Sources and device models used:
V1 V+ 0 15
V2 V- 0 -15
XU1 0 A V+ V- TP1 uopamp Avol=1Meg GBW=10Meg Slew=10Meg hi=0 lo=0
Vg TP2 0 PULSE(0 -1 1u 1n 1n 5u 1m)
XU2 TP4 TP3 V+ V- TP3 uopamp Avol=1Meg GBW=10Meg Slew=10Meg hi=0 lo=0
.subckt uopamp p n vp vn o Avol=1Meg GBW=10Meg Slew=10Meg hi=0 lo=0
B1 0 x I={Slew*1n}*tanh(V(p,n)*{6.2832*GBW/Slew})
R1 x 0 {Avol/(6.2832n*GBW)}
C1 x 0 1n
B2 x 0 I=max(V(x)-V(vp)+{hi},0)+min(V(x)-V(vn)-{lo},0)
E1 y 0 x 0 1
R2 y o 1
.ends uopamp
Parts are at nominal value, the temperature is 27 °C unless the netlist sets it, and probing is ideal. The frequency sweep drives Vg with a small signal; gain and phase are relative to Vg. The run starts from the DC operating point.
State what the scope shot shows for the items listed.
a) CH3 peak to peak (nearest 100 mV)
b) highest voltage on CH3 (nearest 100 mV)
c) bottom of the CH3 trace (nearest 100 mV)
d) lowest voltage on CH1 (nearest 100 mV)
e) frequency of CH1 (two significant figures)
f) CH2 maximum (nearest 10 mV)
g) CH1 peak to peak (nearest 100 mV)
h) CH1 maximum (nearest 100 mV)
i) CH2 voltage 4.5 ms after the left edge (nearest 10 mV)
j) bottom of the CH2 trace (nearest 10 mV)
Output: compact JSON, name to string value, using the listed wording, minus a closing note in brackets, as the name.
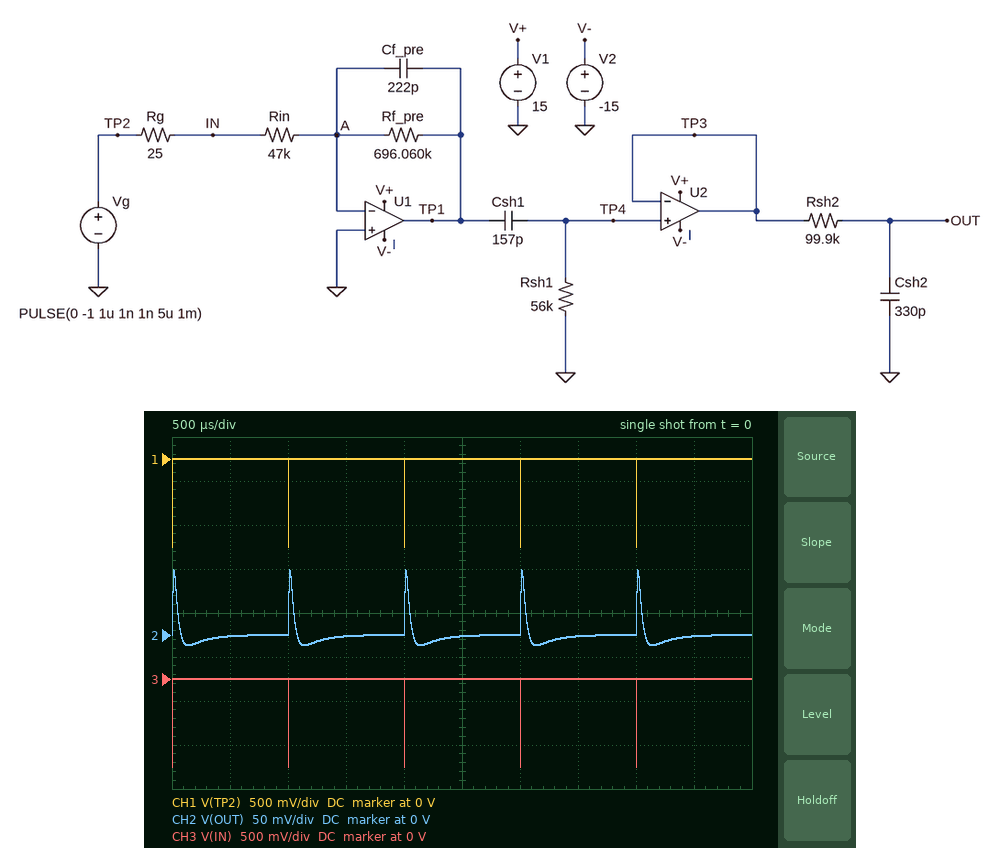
{"CH3 peak to peak": "1.0 V", "highest voltage on CH3": "0 V", "bottom of the CH3 trace": "-1.0 V", "lowest voltage on CH1": "-1.0 V", "frequency of CH1": "1.0 kHz", "CH2 maximum": "70 mV", "CH1 peak to peak": "1.0 V", "CH1 maximum": "0 V", "CH2 voltage 4.5 ms after the left edge": "0 V", "bottom of the CH2 trace": "-10 mV"}
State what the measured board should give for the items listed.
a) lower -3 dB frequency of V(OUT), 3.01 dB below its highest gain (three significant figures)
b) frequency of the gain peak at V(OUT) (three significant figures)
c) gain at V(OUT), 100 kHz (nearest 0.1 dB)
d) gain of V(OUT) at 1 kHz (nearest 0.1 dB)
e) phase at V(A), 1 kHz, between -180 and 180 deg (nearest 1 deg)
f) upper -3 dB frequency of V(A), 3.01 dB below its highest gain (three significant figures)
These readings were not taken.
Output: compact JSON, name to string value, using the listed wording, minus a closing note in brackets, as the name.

{"lower -3 dB frequency of V(OUT), 3.01 dB below its highest gain": "744 Hz", "frequency of the gain peak at V(OUT)": "2.17 kHz", "gain at V(OUT), 100 kHz": "-42.8 dB", "gain of V(OUT) at 1 kHz": "-4.8 dB", "phase at V(A), 1 kHz, between -180 and 180 deg": "45 deg", "upper -3 dB frequency of V(A), 3.01 dB below its highest gain": "10.0 MHz"}
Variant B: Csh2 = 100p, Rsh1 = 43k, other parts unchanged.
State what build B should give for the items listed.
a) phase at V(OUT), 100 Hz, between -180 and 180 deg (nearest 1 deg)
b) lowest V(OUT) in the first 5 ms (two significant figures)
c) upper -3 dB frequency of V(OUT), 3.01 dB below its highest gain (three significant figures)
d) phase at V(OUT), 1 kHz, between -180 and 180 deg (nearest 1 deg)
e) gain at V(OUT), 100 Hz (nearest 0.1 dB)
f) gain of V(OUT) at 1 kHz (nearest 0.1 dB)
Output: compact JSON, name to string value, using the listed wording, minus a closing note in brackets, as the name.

{"phase at V(OUT), 100 Hz, between -180 and 180 deg": "-96 deg", "lowest V(OUT) in the first 5 ms": "-14 mV", "upper -3 dB frequency of V(OUT), 3.01 dB below its highest gain": "13.6 kHz", "phase at V(OUT), 1 kHz, between -180 and 180 deg": "-140 deg", "gain at V(OUT), 100 Hz": "-24.1 dB", "gain of V(OUT) at 1 kHz": "-7.0 dB"}
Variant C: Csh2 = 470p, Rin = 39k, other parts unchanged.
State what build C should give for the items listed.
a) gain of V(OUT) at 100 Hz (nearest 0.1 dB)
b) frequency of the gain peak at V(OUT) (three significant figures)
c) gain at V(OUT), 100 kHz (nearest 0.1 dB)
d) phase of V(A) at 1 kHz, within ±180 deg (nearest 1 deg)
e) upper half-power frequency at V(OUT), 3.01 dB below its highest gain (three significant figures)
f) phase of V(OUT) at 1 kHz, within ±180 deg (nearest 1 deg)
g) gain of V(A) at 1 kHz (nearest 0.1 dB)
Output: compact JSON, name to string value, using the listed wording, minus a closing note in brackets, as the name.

{"gain of V(OUT) at 100 Hz": "-20.2 dB", "frequency of the gain peak at V(OUT)": "1.84 kHz", "gain at V(OUT), 100 kHz": "-44.3 dB", "phase of V(A) at 1 kHz, within ±180 deg": "45 deg", "upper half-power frequency at V(OUT), 3.01 dB below its highest gain": "4.87 kHz", "phase of V(OUT) at 1 kHz, within ±180 deg": "-154 deg", "gain of V(A) at 1 kHz": "-57.9 dB"}
